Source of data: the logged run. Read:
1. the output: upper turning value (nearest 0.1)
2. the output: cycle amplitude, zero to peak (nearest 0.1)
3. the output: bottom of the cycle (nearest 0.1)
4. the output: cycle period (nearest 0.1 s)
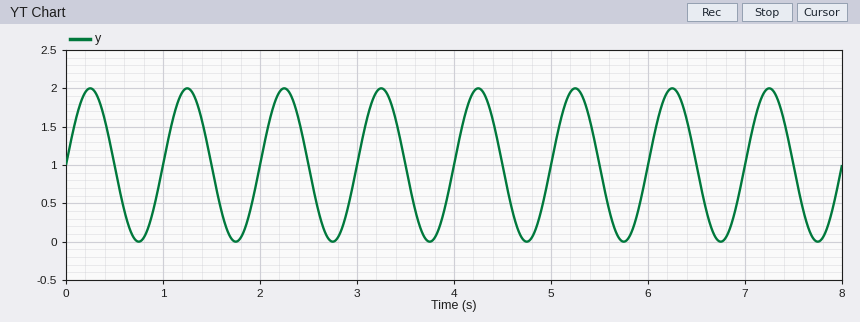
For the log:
2.0
1.0
0.0
1.0 s
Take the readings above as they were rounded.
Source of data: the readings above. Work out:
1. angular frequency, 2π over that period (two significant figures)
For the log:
6.3 rad/s
